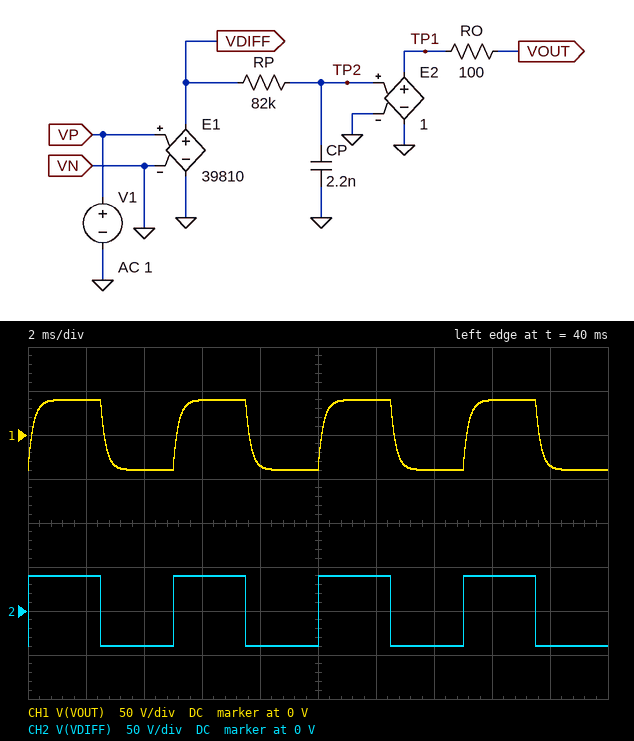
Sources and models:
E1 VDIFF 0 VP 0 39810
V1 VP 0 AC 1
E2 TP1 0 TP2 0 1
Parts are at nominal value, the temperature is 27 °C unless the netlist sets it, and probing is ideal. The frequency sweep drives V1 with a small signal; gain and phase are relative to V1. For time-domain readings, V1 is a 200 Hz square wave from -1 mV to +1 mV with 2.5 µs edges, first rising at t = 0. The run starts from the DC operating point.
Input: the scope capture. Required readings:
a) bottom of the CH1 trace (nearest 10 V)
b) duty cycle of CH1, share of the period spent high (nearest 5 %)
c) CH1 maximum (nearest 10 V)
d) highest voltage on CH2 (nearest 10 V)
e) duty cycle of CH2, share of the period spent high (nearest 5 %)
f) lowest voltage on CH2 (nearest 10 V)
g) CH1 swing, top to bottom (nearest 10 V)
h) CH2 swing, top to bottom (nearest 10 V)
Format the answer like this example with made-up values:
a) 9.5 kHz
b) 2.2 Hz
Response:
a) -40 V
b) 50 %
c) 40 V
d) 40 V
e) 50 %
f) -40 V
g) 80 V
h) 80 V
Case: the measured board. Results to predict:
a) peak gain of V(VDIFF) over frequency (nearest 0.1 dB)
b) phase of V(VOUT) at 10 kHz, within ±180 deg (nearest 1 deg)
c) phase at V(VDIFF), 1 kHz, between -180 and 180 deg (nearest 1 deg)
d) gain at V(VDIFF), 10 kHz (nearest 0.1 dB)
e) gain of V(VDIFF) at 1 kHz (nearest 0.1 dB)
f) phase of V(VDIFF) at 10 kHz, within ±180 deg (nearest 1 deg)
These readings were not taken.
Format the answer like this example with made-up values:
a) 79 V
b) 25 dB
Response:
a) 92.0 dB
b) -85 deg
c) 0 deg
d) 92.0 dB
e) 92.0 dB
f) 0 deg
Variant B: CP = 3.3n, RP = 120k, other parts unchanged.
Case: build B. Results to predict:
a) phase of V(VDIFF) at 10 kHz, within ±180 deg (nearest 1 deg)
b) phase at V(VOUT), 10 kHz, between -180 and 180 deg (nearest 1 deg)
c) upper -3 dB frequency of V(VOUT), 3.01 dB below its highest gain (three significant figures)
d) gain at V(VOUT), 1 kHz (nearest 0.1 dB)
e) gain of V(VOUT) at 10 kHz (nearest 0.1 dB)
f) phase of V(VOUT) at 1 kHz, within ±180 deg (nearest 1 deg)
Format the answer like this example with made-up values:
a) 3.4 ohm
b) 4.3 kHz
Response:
a) 0 deg
b) -88 deg
c) 402 Hz
d) 83.4 dB
e) 64.1 dB
f) -68 deg
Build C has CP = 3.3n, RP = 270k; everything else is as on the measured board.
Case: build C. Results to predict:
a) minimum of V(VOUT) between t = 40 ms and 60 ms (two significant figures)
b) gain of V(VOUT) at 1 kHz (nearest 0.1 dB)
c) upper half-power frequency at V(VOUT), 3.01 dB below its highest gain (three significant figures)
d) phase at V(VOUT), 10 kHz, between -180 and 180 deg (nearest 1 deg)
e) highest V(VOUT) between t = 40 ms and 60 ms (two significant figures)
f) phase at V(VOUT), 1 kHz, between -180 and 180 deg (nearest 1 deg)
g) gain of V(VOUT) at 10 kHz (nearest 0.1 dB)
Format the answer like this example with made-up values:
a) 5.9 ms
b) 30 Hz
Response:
a) -35 V
b) 76.9 dB
c) 179 Hz
d) -89 deg
e) 35 V
f) -80 deg
g) 57.0 dB
